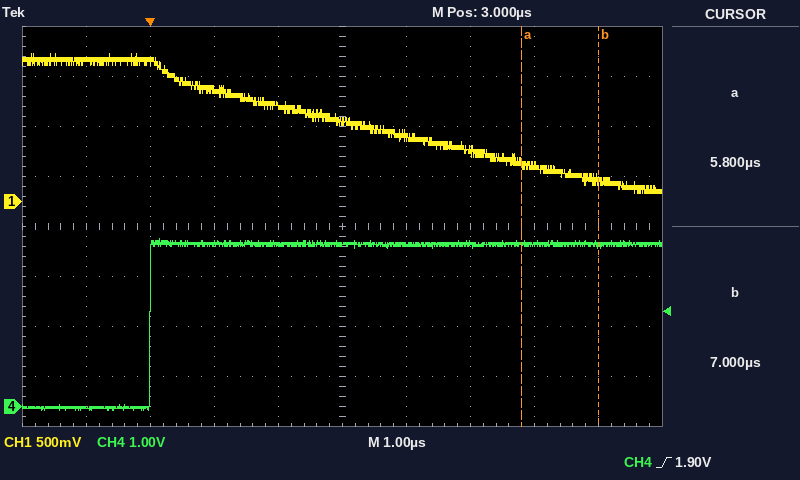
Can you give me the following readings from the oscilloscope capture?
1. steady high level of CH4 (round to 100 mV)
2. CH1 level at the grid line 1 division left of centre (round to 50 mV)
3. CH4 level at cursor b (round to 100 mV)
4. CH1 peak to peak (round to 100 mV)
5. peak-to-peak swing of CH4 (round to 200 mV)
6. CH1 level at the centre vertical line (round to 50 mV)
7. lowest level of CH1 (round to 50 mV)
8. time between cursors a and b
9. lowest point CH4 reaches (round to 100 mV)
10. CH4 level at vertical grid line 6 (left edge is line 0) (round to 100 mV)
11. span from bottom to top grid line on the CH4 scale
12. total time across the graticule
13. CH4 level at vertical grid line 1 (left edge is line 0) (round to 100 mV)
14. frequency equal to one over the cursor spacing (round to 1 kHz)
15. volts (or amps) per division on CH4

3.2 V
950 mV
3.2 V
1.40 V
3.4 V
800 mV
100 mV
1.2 µs
-100 mV
3.2 V
8 V
10 µs
0.0 V
833 kHz
1 V
